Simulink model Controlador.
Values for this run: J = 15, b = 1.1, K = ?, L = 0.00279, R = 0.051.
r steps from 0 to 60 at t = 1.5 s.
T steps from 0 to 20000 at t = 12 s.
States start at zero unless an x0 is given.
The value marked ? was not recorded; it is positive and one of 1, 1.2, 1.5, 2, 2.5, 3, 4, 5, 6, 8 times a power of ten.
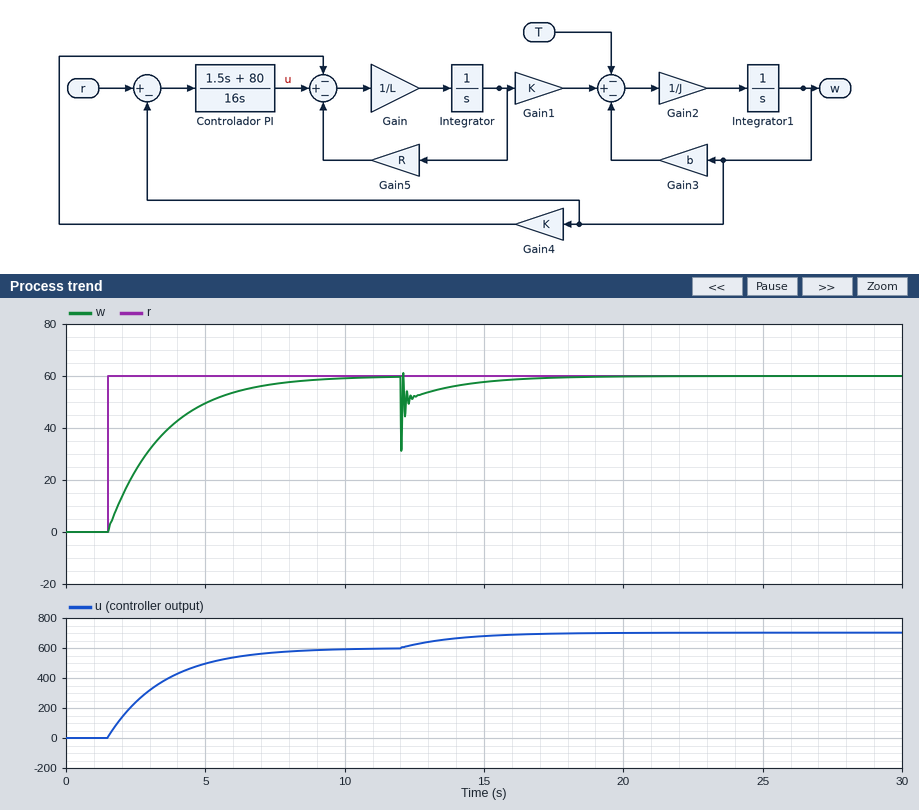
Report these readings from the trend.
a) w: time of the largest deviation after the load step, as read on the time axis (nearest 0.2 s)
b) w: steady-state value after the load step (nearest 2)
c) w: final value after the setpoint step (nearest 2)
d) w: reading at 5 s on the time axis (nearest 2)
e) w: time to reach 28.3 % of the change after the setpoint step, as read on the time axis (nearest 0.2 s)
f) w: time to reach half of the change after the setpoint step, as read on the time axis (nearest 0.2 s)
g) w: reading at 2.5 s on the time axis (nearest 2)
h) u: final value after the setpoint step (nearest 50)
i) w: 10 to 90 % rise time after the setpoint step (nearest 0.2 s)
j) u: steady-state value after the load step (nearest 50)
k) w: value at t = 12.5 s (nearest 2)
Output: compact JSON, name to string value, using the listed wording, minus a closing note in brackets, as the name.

{"w: time of the largest deviation after the load step, as read on the time axis": "12.0 s", "w: steady-state value after the load step": "60", "w: final value after the setpoint step": "60", "w: reading at 5 s on the time axis": "50", "w: time to reach 28.3 % of the change after the setpoint step, as read on the time axis": "2.2 s", "w: time to reach half of the change after the setpoint step, as read on the time axis": "2.8 s", "w: reading at 2.5 s on the time axis": "24", "u: final value after the setpoint step": "600", "w: 10 to 90 % rise time after the setpoint step": "4.4 s", "u: steady-state value after the load step": "700", "w: value at t = 12.5 s": "52"}
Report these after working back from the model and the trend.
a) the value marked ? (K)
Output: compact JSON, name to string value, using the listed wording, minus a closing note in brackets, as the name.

{"the value marked ?": "10"}
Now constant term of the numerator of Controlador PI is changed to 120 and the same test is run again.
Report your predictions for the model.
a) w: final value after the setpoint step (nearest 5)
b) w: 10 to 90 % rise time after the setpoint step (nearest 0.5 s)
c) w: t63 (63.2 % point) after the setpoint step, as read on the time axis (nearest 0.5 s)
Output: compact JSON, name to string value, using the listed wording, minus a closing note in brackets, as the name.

{"w: final value after the setpoint step": "60", "w: 10 to 90 % rise time after the setpoint step": "3.0 s", "w: t63 (63.2 % point) after the setpoint step, as read on the time axis": "3.0 s"}
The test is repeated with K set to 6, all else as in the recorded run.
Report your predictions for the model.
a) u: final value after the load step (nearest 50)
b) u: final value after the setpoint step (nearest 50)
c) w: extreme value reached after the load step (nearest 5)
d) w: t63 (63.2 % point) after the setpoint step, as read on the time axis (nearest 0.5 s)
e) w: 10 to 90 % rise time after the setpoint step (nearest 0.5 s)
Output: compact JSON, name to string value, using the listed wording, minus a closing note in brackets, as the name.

{"u: final value after the load step": "550", "u: final value after the setpoint step": "350", "w: extreme value reached after the load step": "10", "w: t63 (63.2 % point) after the setpoint step, as read on the time axis": "2.5 s", "w: 10 to 90 % rise time after the setpoint step": "2.5 s"}
